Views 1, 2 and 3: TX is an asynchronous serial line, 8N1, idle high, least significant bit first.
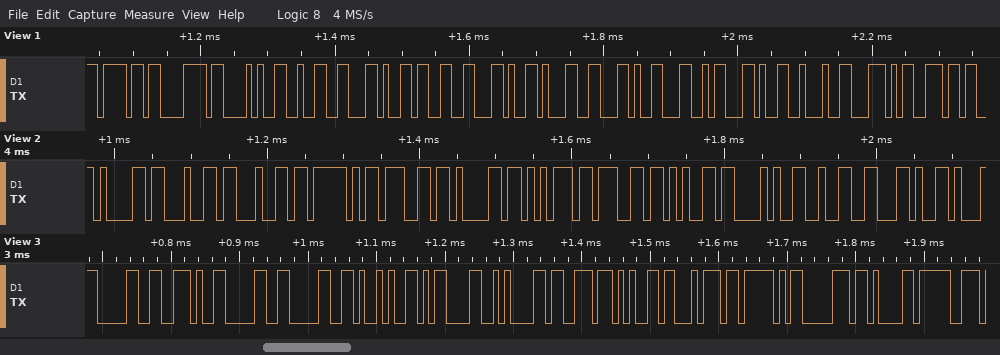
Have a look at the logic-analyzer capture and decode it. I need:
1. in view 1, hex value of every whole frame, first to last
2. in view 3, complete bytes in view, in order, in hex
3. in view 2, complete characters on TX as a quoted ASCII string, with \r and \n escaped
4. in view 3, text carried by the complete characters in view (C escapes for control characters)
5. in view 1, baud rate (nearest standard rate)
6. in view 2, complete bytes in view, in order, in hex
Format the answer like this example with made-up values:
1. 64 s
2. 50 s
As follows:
1. 6F 78 28 32 2C 33 2C 31 2C 4C 2C 22 5C 6E
2. 30 2E 30 30 29 0D 0A 73 65 74 5F 70 61
3. "add_gauge(2,"
4. "0.00)\r\nset_pa"
5. 115200 baud
6. 0x61 0x64 0x64 0x5F 0x67 0x61 0x75 0x67 0x65 0x28 0x32 0x2C
